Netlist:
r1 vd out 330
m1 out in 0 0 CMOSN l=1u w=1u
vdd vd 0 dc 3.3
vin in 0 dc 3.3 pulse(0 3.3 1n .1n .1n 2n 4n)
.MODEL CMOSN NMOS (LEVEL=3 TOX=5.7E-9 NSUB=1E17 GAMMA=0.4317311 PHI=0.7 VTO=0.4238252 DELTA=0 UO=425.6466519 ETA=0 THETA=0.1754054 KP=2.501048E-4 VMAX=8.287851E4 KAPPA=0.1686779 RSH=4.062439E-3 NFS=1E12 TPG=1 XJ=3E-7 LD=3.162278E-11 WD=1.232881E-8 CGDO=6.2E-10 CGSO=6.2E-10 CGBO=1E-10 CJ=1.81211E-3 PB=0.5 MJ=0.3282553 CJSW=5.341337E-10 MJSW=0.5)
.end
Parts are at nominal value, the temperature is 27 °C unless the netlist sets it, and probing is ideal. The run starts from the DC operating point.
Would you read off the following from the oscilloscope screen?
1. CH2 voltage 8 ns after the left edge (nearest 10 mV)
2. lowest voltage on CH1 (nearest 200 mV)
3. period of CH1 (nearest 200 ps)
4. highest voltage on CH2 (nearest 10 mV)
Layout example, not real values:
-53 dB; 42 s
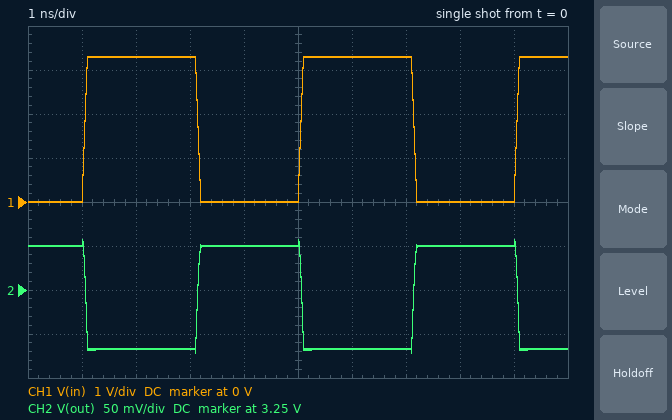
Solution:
3.30 V; 0 V; 4.0 ns; 3.31 V
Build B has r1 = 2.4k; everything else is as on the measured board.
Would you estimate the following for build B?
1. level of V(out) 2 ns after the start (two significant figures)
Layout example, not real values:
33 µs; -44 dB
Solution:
2.5 V
